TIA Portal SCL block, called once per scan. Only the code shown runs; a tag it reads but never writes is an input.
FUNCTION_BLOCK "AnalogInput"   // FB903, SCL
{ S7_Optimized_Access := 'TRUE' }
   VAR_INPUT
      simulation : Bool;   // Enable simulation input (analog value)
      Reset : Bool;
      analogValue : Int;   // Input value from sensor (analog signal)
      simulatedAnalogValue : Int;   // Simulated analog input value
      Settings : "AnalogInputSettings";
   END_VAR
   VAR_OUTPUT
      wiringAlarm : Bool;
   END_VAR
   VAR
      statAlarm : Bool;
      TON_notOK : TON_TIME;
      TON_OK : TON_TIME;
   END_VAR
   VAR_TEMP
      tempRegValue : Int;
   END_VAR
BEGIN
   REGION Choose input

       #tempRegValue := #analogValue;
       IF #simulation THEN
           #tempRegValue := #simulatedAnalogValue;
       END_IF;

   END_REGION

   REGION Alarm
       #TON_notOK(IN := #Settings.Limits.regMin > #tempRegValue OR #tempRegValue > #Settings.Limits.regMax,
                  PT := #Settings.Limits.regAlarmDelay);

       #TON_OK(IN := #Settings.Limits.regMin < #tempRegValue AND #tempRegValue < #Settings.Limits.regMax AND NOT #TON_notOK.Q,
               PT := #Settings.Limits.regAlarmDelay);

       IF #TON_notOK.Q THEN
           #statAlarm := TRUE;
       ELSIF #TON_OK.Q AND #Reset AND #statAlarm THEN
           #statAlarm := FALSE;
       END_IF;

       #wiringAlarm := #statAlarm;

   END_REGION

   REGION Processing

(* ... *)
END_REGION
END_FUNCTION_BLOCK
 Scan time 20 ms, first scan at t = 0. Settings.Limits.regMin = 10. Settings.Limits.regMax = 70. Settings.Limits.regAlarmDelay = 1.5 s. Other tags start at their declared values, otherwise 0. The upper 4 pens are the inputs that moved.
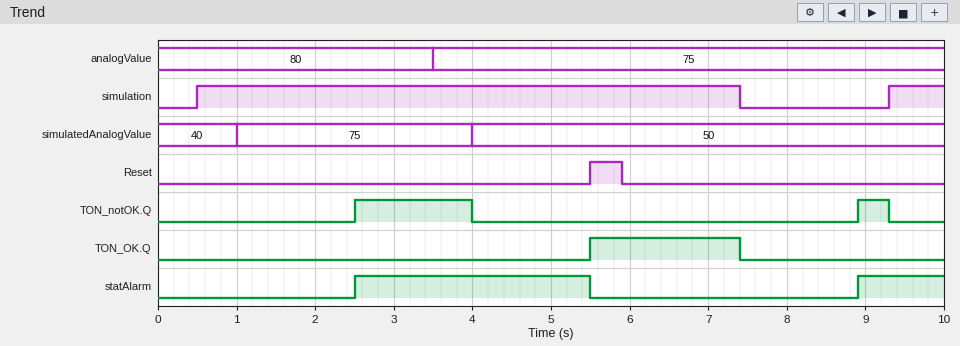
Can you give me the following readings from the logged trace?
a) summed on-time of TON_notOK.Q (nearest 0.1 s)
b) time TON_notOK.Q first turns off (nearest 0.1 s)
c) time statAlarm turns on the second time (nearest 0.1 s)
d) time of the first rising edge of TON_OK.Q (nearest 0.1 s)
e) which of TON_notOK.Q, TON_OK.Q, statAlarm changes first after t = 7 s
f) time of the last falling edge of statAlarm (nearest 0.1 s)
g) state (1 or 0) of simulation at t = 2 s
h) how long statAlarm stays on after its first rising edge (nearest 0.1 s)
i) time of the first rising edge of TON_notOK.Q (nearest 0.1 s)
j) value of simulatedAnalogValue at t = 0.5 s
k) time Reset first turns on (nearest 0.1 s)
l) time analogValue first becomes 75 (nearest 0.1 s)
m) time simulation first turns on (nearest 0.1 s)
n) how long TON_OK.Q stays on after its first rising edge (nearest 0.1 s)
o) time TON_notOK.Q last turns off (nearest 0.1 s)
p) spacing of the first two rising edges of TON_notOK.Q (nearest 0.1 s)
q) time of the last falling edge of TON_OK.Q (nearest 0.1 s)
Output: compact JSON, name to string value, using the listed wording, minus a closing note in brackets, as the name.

{"summed on-time of TON_notOK.Q": "1.9 s", "time TON_notOK.Q first turns off": "4.0 s", "time statAlarm turns on the second time": "8.9 s", "time of the first rising edge of TON_OK.Q": "5.5 s", "which of TON_notOK.Q, TON_OK.Q, statAlarm changes first after t = 7 s": "TON_OK.Q", "time of the last falling edge of statAlarm": "5.5 s", "state (1 or 0) of simulation at t = 2 s": "1", "how long statAlarm stays on after its first rising edge": "3.0 s", "time of the first rising edge of TON_notOK.Q": "2.5 s", "value of simulatedAnalogValue at t = 0.5 s": "40", "time Reset first turns on": "5.5 s", "time analogValue first becomes 75": "3.5 s", "time simulation first turns on": "0.5 s", "how long TON_OK.Q stays on after its first rising edge": "1.9 s", "time TON_notOK.Q last turns off": "9.3 s", "spacing of the first two rising edges of TON_notOK.Q": "6.4 s", "time of the last falling edge of TON_OK.Q": "7.4 s"}
